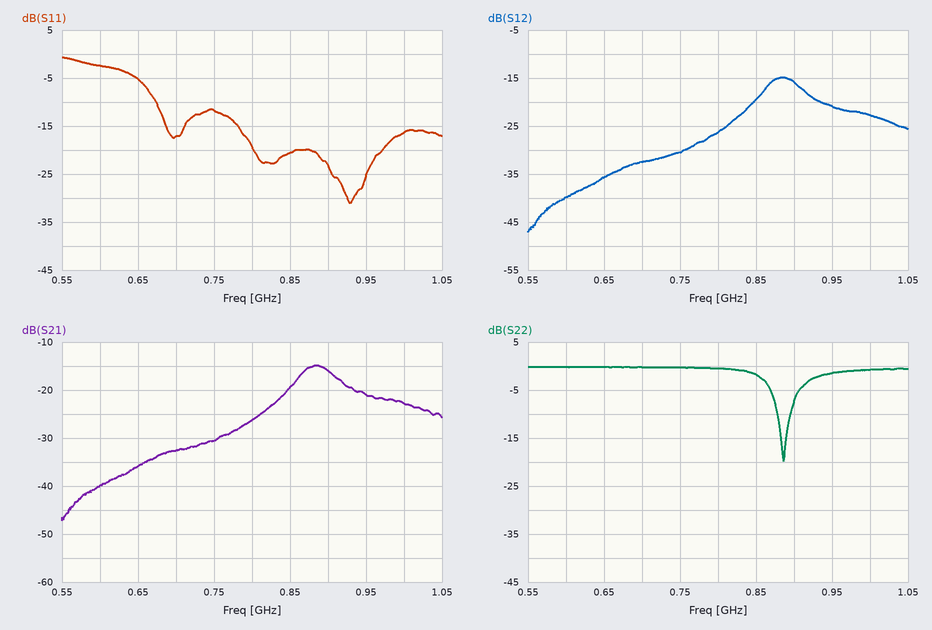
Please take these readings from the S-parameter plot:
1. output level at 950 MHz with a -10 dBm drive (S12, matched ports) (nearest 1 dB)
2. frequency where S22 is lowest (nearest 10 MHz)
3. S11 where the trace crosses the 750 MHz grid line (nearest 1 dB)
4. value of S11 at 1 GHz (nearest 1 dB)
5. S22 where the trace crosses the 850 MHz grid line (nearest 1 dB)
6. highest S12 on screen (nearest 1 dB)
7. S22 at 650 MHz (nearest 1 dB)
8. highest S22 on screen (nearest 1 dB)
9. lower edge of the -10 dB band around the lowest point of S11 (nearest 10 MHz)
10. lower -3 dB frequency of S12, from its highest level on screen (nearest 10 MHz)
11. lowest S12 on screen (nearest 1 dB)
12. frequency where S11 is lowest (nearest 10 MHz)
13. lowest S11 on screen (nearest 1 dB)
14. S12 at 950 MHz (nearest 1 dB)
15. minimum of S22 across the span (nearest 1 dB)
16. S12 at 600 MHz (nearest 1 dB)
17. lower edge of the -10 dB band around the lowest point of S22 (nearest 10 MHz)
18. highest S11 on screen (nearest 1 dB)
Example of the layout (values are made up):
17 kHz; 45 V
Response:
-31 dBm; 890 MHz; -12 dB; -16 dB; -2 dB; -15 dB; 0 dB; 0 dB; 670 MHz; 860 MHz; -47 dB; 930 MHz; -31 dB; -21 dB; -20 dB; -40 dB; 880 MHz; -1 dB
